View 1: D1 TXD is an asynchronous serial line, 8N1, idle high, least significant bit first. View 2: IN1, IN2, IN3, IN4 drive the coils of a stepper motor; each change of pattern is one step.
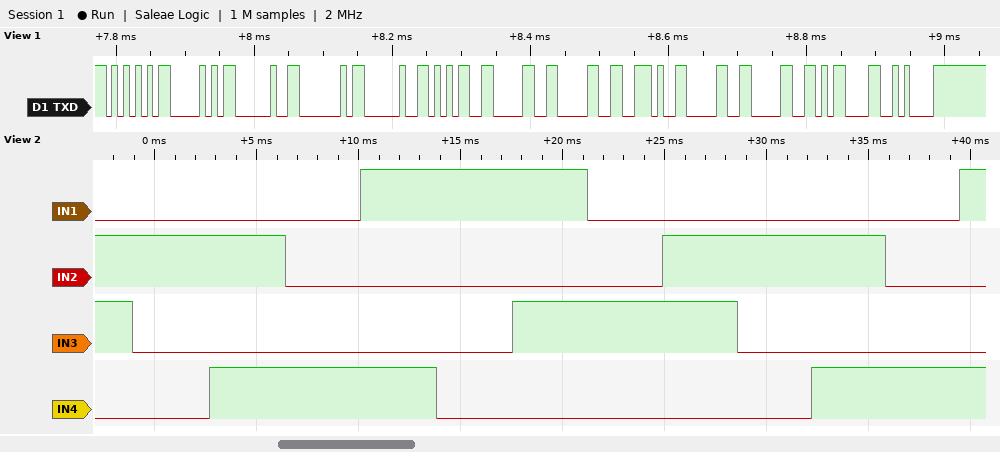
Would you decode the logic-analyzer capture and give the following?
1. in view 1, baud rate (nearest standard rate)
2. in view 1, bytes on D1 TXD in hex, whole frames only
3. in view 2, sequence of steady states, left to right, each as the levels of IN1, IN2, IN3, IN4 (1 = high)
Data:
115200 baud
0x55 0x50 0x20 0x40 0x20 0x35 0x30 0x30 0x2E 0x30 0x30 0x0D 0x0A
0110 0100 0101 0001 1001 1000 1010 0010 0110 0100 0101 0001 1001
